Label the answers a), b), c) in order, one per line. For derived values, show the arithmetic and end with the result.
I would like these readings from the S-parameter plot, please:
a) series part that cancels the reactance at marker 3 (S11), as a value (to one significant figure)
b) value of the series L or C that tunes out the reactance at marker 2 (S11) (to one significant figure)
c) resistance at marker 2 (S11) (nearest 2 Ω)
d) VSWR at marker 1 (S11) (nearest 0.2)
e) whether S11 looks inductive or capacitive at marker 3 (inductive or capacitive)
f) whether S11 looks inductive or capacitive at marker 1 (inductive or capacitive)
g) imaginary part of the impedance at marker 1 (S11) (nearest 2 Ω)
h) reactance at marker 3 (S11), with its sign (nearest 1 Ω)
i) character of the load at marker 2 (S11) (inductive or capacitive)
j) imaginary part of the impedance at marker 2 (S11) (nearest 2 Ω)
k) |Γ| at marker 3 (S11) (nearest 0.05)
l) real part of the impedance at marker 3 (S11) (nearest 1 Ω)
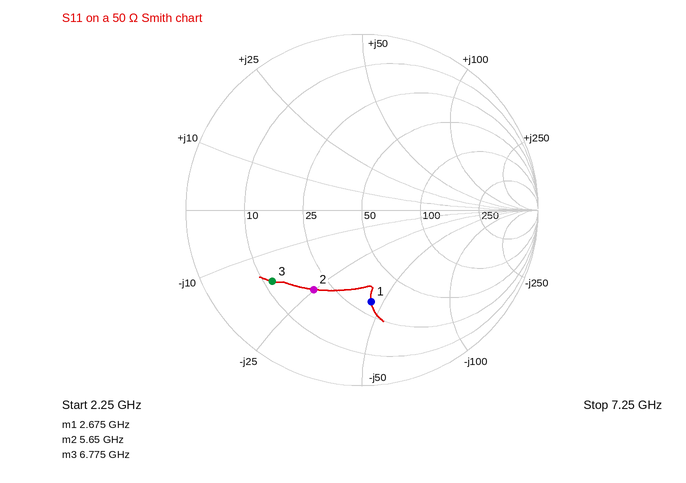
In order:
a) L = 17 Ω/(2π × 6.775 GHz) ≈ 399 pH, so 400 pH to one significant figure
b) L = 24 Ω/(2π × 5.65 GHz) ≈ 676 pH, so 700 pH to one significant figure
c) 20 Ω
d) 3.2
e) capacitive
f) capacitive
g) -44 Ω
h) -17 Ω
i) capacitive
j) -24 Ω
k) 0.65
l) 12 Ω
